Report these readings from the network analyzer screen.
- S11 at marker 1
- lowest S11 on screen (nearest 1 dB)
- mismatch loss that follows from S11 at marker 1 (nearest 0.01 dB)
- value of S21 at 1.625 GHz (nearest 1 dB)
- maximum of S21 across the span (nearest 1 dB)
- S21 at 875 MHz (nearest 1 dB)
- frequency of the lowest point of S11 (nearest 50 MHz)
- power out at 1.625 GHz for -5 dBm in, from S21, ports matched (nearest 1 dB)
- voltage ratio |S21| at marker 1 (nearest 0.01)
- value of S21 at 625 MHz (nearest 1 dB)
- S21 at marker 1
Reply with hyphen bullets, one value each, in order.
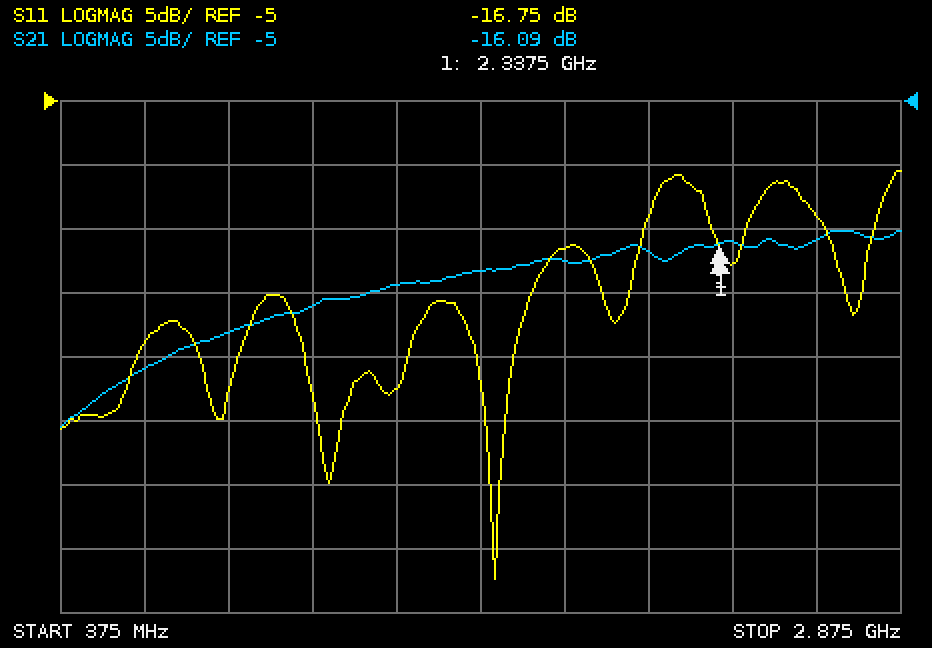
- -16.75 dB
- -42 dB
- 0.09 dB
- -18 dB
- -15 dB
- -23 dB
- 1.65 GHz
- -23 dBm
- 0.16
- -26 dB
- -16.09 dB
